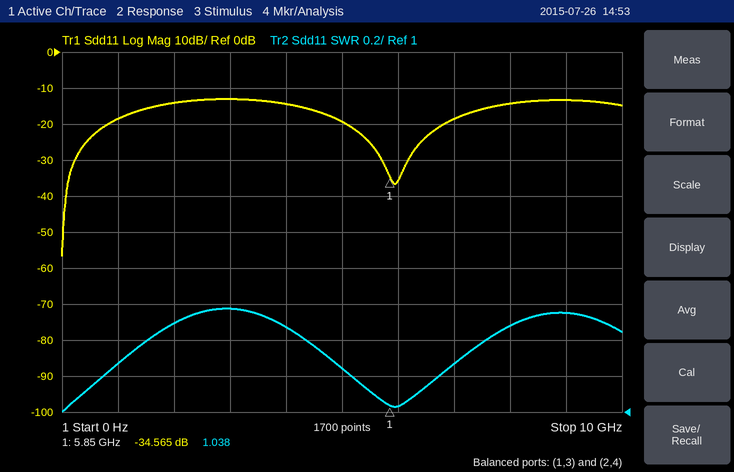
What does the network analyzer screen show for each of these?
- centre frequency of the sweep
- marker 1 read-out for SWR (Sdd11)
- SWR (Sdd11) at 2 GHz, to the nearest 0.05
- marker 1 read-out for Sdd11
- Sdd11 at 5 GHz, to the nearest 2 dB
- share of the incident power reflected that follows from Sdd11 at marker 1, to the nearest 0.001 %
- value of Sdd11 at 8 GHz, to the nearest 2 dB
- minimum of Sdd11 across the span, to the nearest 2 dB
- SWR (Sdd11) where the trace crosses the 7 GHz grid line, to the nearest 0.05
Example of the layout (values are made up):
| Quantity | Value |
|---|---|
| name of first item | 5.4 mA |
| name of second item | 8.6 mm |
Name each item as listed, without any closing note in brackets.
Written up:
| Quantity | Value |
|---|---|
| centre frequency of the sweep | 5 GHz |
| marker 1 read-out for SWR | 1.038 |
| SWR (Sdd11) at 2 GHz, to the nearest 0.05 | 1.50 |
| marker 1 read-out for Sdd11 | -34.565 dB |
| Sdd11 at 5 GHz, to the nearest 2 dB | -20 dB |
| share of the incident power reflected that follows from Sdd11 at marker 1, to the nearest 0.001 % | 0.035 % |
| value of Sdd11 at 8 GHz, to the nearest 2 dB | -14 dB |
| minimum of Sdd11 across the span, to the nearest 2 dB | -56 dB |
| SWR (Sdd11) where the trace crosses the 7 GHz grid line, to the nearest 0.05 | 1.25 |
